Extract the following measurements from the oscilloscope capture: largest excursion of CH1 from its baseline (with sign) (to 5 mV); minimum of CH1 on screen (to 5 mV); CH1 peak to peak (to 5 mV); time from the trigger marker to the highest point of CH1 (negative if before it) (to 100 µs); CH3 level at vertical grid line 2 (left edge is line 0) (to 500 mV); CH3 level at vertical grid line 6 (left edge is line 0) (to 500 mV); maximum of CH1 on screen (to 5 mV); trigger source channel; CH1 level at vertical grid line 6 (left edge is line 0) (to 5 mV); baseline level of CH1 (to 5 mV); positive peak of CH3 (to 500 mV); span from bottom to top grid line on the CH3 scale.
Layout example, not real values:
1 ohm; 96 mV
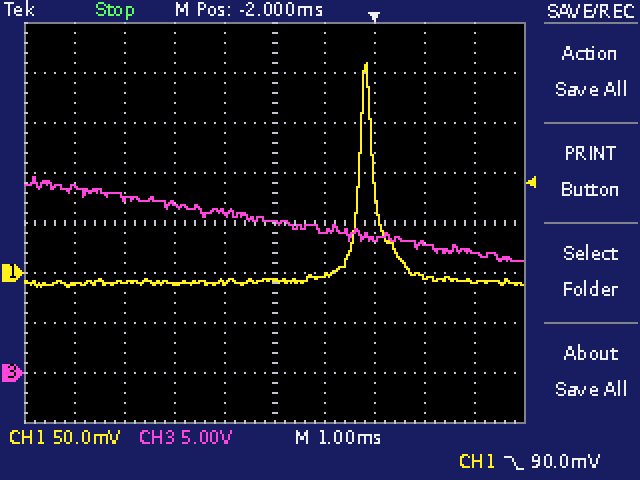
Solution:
+220 mV; -15 mV; 225 mV; -200 µs; 17.5 V; 14.0 V; 210 mV; CH1; 0 mV; -10 mV; 19.5 V; 40 V
